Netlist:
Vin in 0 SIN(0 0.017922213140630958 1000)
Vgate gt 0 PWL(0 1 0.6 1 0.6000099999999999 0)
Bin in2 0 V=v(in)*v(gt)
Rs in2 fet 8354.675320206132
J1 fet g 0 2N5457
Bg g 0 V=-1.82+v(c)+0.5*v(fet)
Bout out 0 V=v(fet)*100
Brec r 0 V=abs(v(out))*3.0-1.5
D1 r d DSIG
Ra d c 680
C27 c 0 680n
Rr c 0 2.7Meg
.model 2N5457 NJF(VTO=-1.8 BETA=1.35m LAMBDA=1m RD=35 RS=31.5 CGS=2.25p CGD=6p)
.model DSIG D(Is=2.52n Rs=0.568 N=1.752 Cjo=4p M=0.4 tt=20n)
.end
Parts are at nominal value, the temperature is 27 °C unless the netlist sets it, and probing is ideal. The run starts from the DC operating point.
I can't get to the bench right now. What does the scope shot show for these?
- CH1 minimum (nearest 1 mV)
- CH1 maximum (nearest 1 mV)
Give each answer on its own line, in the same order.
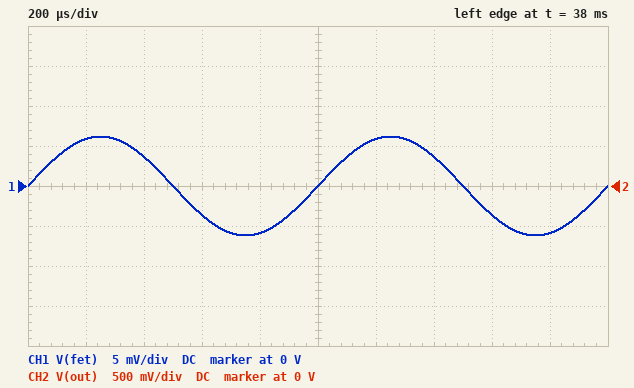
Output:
-6 mV
6 mV
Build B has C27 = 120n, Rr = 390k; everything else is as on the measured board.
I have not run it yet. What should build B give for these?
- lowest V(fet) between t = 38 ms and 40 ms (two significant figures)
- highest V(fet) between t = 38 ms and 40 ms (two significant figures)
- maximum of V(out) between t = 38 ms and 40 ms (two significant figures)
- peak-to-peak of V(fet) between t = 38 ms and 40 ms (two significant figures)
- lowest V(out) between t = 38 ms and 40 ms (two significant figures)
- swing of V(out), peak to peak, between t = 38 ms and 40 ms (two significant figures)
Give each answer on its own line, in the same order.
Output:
-6.4 mV
6.4 mV
640 mV
13 mV
-640 mV
1.3 V
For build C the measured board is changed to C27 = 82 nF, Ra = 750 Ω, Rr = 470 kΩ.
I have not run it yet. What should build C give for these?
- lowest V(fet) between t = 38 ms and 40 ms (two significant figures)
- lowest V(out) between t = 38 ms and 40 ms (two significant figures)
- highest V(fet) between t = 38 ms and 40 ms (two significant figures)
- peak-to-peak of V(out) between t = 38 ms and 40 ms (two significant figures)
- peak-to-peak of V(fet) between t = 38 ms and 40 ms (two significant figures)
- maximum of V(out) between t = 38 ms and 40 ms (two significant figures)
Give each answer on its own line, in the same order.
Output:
-6.3 mV
-630 mV
6.3 mV
1.3 V
13 mV
630 mV
